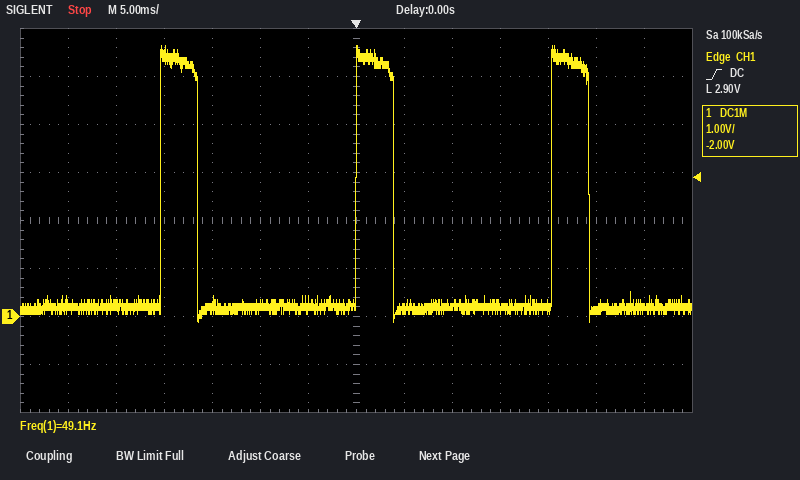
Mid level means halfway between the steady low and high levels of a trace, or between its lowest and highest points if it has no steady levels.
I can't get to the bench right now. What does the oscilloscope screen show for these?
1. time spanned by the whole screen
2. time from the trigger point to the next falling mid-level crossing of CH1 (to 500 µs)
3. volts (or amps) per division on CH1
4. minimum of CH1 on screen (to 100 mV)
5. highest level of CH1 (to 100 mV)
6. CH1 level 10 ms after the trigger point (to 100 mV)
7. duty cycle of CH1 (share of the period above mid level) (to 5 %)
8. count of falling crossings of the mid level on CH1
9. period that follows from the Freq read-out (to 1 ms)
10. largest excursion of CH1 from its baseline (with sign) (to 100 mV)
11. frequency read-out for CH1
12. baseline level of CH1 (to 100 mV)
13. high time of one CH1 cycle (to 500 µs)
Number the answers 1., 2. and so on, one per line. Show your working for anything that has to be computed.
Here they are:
1. 70 ms
2. 4.0 ms
3. 1 V
4. -100 mV
5. 5.6 V
6. 200 mV
7. 20 %
8. 3
9. 1 / 49.1 Hz ≈ 20 ms
10. 5.6 V − (200 mV) = +5.4 V
11. 49.1 Hz
12. 200 mV
13. 4.0 ms
